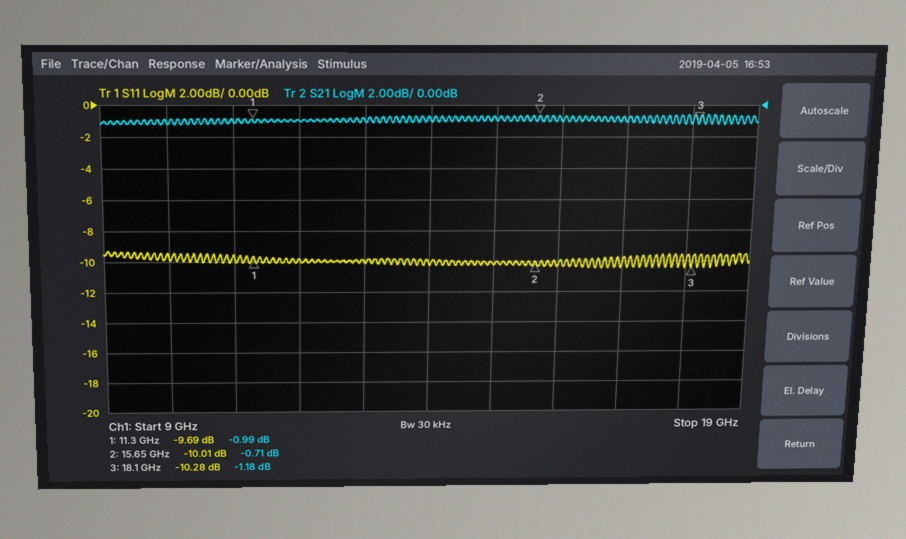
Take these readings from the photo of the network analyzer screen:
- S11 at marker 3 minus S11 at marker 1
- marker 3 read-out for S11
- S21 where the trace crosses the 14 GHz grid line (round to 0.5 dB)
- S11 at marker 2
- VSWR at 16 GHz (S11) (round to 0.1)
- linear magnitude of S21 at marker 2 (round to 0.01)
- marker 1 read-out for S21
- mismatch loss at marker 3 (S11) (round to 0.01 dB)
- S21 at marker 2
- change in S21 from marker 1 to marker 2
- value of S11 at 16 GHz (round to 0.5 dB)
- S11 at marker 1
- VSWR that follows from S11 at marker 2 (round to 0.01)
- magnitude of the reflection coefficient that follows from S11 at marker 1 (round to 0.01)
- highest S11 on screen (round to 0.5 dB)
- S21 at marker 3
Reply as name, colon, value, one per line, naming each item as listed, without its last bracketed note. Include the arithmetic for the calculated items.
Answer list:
S11 at marker 3 minus S11 at marker 1: -10.28 − (-9.69) = -0.59 dB
marker 3 read-out for S11: -10.28 dB
S21 where the trace crosses the 14 GHz grid line: -1.0 dB
S11 at marker 2: -10.01 dB
VSWR at 16 GHz (S11): |Γ| = 10^(-10.5/20) = 0.2985; VSWR = (1 + 0.2985)/(1 − 0.2985) ≈ 1.9
linear magnitude of S21 at marker 2: 10^(-0.71/20) ≈ 0.92
marker 1 read-out for S21: -0.99 dB
mismatch loss at marker 3 (S11): −10 log10(1 − 10^(-10.28/10)) ≈ 0.43 dB
S21 at marker 2: -0.71 dB
change in S21 from marker 1 to marker 2: -0.71 − (-0.99) = 0.28 dB
value of S11 at 16 GHz: -10.5 dB
S11 at marker 1: -9.69 dB
VSWR that follows from S11 at marker 2: (1 + 0.3159)/(1 − 0.3159) ≈ 1.92
magnitude of the reflection coefficient that follows from S11 at marker 1: 10^(-9.69/20) ≈ 0.33
highest S11 on screen: -9.5 dB
S21 at marker 3: -1.18 dB
